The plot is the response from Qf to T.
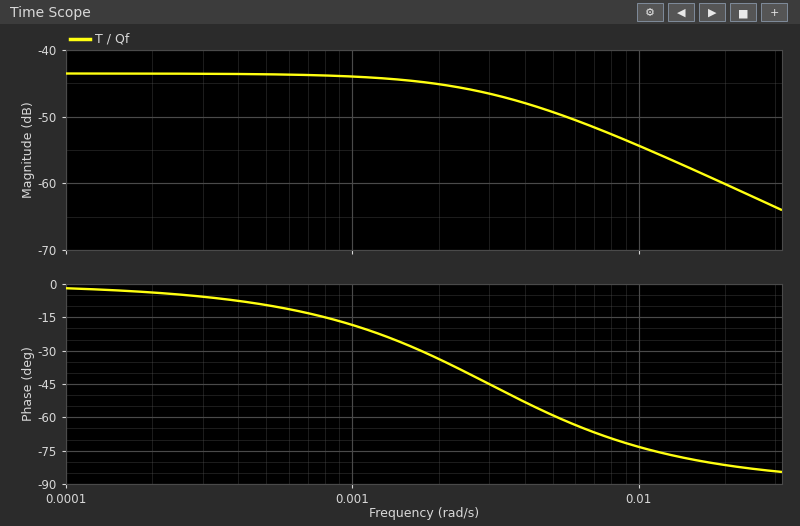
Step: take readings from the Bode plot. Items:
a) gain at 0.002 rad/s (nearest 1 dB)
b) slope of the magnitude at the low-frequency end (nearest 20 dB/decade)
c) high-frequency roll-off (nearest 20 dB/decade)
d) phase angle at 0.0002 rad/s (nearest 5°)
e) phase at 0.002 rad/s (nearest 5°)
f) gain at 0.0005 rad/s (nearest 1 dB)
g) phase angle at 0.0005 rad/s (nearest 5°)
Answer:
-45 dB
0 dB/decade
-20 dB/decade
-5°
-35°
-44 dB
-10°
